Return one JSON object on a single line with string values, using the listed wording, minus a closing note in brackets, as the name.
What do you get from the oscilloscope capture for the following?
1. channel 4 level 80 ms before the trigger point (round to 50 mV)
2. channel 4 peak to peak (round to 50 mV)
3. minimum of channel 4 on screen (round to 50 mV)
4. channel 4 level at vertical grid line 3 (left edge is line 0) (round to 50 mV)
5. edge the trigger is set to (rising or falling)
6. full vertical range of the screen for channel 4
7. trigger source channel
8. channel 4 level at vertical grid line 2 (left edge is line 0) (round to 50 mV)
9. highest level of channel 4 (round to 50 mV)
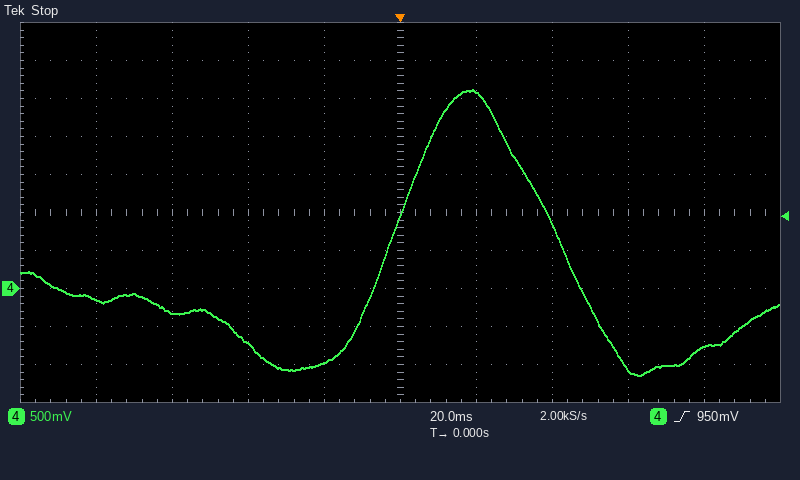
{"channel 4 level 80 ms before the trigger point": "-150 mV", "channel 4 peak to peak": "3.75 V", "minimum of channel 4 on screen": "-1.15 V", "channel 4 level at vertical grid line 3 (left edge is line 0)": "-750 mV", "edge the trigger is set to": "rising", "full vertical range of the screen for channel 4": "5 V", "trigger source channel": "channel 4", "channel 4 level at vertical grid line 2 (left edge is line 0)": "-300 mV", "highest level of channel 4": "2.60 V"}
